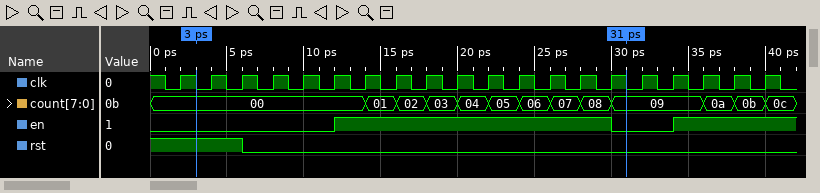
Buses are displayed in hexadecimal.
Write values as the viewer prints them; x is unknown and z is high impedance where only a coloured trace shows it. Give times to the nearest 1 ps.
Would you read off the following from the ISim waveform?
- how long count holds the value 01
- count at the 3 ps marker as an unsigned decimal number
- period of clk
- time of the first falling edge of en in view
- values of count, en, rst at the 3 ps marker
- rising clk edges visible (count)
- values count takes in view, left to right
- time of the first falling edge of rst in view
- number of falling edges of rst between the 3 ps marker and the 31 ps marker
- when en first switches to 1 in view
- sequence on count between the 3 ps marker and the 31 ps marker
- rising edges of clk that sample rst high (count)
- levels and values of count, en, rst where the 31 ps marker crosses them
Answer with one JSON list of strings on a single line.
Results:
["2 ps", "0", "2 ps", "30 ps", "count=00, en=0, rst=1", "20", "00, 01, 02, 03, 04, 05, 06, 07, 08, 09, 0a, 0b, 0c", "6 ps", "1", "12 ps", "00, 01, 02, 03, 04, 05, 06, 07, 08, 09", "3", "count=09, en=0, rst=0"]
